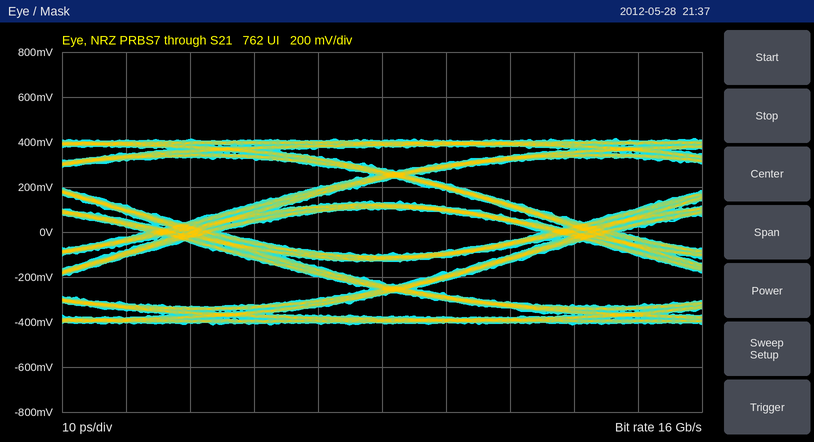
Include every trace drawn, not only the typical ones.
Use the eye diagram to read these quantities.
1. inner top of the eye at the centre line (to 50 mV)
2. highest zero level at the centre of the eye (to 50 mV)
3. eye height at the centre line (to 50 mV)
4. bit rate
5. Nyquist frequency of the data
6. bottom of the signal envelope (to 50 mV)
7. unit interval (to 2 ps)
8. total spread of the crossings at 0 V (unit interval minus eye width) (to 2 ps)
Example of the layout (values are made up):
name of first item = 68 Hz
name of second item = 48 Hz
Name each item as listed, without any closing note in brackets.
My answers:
inner top of the eye at the centre line = 100 mV
highest zero level at the centre of the eye = -100 mV
eye height at the centre line = 200 mV
bit rate = 16 Gb/s
Nyquist frequency of the data = 8 GHz
bottom of the signal envelope = -400 mV
unit interval = 62 ps
total spread of the crossings at 0 V (unit interval minus eye width) = 12 ps
